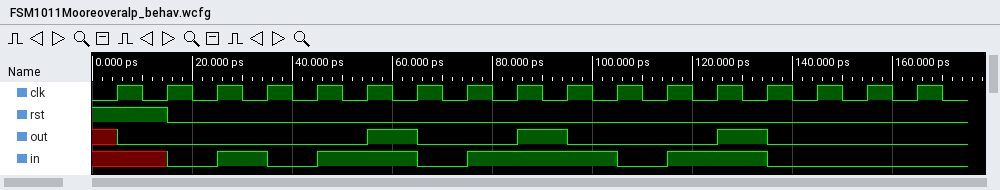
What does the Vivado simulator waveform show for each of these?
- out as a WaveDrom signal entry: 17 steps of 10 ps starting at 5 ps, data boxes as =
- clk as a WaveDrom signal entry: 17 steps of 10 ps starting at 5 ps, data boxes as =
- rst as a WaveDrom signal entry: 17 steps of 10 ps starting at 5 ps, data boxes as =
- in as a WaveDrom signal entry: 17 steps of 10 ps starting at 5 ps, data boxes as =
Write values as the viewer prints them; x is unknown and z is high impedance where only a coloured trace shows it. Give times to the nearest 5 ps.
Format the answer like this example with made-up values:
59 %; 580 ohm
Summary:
{name: 'out', wave: '0....10.10..10...'}; {name: 'clk', wave: 'p................'}; {name: 'rst', wave: '10...............'}; {name: 'in', wave: 'x0101.01..01.0...'}
